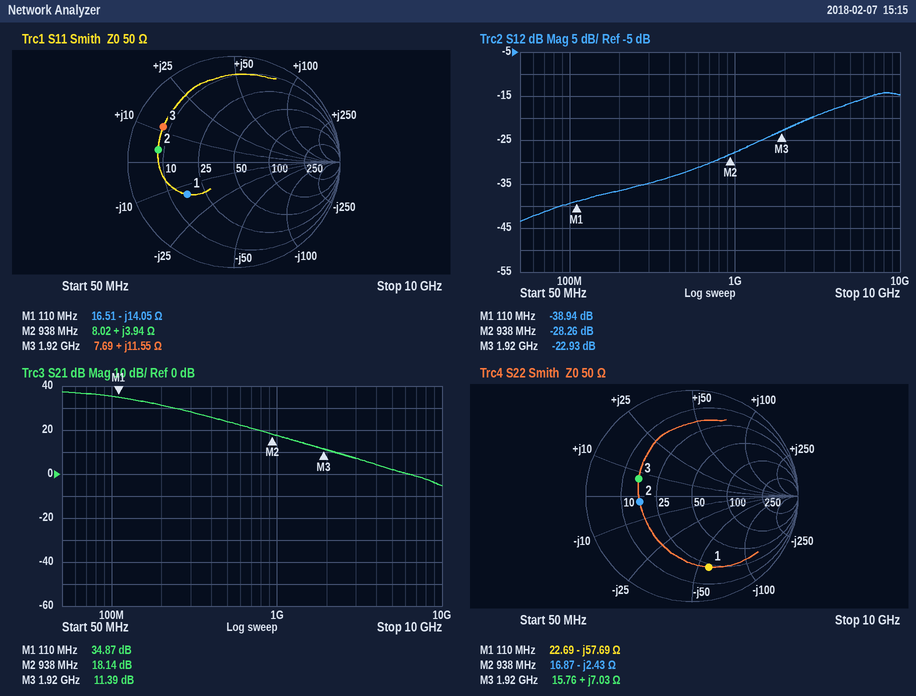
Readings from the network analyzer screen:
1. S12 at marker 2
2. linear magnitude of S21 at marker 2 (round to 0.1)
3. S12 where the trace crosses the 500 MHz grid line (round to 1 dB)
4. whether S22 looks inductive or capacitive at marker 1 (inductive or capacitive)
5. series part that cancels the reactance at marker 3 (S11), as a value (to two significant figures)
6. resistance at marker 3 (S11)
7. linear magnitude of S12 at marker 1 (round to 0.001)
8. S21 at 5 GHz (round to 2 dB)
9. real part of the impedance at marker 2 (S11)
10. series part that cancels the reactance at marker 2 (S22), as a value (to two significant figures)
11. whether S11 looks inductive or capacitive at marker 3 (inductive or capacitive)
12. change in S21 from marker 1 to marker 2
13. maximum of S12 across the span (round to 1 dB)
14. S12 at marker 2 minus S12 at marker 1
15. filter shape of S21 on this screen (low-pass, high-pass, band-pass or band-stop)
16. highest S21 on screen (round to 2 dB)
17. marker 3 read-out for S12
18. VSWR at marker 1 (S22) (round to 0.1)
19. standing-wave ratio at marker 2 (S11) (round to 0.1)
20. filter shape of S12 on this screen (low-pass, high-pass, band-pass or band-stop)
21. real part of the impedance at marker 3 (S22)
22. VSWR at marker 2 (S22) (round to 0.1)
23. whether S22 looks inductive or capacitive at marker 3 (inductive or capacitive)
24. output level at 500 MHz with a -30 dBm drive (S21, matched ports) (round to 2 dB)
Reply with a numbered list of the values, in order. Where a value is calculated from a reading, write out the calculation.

1. -28.26 dB
2. 10^(18.14/20) ≈ 8.1
3. -32 dB
4. capacitive
5. C = 1/(2π × 1.92 GHz × 11.55 Ω) ≈ 7.2 pF
6. 7.69 Ω
7. 10^(-38.94/20) ≈ 0.011
8. 2 dB
9. 8.02 Ω
10. L = 2.43 Ω/(2π × 938 MHz) ≈ 412 pH, so 410 pH to two significant figures
11. inductive
12. 18.14 − (34.87) = -16.73 dB
13. -14 dB
14. -28.26 − (-38.94) = 10.68 dB
15. low-pass
16. 38 dB
17. -22.93 dB
18. 5.4
19. 6.3
20. high-pass
21. 15.76 Ω
22. 3.0
23. inductive
24. -30 dBm + (24 dB) = -6 dBm
